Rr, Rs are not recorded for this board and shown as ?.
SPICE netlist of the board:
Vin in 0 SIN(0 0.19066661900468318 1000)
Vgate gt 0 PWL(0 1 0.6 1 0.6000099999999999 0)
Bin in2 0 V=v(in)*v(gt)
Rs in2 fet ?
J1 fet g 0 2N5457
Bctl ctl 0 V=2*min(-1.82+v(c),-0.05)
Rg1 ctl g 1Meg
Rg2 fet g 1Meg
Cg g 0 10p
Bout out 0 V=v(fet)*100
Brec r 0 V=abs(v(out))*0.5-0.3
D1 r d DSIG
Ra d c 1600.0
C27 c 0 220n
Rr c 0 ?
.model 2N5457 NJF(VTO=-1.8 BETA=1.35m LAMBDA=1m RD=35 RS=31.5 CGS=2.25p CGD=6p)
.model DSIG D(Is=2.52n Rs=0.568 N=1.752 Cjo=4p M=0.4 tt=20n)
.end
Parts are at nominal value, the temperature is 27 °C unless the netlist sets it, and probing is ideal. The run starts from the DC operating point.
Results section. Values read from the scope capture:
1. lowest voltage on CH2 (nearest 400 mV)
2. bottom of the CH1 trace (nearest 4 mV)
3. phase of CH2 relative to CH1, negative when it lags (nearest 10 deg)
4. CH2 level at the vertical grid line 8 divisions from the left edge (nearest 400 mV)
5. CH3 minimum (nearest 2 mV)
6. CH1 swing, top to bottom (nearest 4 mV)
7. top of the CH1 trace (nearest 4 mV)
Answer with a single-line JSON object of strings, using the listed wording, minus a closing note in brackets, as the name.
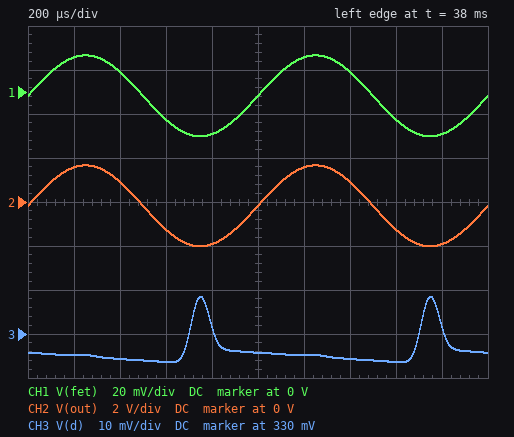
{"lowest voltage on CH2": "-2.0 V", "bottom of the CH1 trace": "-20 mV", "phase of CH2 relative to CH1, negative when it lags": "0 deg", "CH2 level at the vertical grid line 8 divisions from the left edge": "-1.2 V", "CH3 minimum": "324 mV", "CH1 swing, top to bottom": "36 mV", "top of the CH1 trace": "16 mV"}
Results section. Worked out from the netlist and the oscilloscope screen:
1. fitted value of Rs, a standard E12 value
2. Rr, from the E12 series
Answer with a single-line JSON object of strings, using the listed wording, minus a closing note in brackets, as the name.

{"fitted value of Rs, a standard E12 value": "12 kΩ", "Rr, from the E12 series": "390 kΩ"}
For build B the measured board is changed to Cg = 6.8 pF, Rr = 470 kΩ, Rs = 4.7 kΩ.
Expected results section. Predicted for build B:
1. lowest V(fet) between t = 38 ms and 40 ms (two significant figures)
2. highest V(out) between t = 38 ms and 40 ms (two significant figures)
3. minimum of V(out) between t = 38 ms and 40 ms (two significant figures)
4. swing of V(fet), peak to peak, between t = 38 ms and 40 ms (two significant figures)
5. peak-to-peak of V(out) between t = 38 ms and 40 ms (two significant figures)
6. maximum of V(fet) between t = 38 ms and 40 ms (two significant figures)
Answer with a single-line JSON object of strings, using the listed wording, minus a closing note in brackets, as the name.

{"lowest V(fet) between t = 38 ms and 40 ms": "-26 mV", "highest V(out) between t = 38 ms and 40 ms": "2.4 V", "minimum of V(out) between t = 38 ms and 40 ms": "-2.6 V", "swing of V(fet), peak to peak, between t = 38 ms and 40 ms": "50 mV", "peak-to-peak of V(out) between t = 38 ms and 40 ms": "5.0 V", "maximum of V(fet) between t = 38 ms and 40 ms": "24 mV"}
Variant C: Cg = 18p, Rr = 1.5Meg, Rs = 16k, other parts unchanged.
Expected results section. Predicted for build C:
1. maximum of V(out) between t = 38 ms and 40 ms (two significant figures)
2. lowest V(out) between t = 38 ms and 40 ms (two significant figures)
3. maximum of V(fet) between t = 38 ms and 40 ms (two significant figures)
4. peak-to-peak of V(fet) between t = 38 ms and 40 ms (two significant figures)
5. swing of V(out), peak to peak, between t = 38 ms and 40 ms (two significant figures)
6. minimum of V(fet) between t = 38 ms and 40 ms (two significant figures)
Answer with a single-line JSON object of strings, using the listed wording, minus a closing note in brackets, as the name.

{"maximum of V(out) between t = 38 ms and 40 ms": "1.4 V", "lowest V(out) between t = 38 ms and 40 ms": "-1.8 V", "maximum of V(fet) between t = 38 ms and 40 ms": "14 mV", "peak-to-peak of V(fet) between t = 38 ms and 40 ms": "32 mV", "swing of V(out), peak to peak, between t = 38 ms and 40 ms": "3.2 V", "minimum of V(fet) between t = 38 ms and 40 ms": "-18 mV"}
